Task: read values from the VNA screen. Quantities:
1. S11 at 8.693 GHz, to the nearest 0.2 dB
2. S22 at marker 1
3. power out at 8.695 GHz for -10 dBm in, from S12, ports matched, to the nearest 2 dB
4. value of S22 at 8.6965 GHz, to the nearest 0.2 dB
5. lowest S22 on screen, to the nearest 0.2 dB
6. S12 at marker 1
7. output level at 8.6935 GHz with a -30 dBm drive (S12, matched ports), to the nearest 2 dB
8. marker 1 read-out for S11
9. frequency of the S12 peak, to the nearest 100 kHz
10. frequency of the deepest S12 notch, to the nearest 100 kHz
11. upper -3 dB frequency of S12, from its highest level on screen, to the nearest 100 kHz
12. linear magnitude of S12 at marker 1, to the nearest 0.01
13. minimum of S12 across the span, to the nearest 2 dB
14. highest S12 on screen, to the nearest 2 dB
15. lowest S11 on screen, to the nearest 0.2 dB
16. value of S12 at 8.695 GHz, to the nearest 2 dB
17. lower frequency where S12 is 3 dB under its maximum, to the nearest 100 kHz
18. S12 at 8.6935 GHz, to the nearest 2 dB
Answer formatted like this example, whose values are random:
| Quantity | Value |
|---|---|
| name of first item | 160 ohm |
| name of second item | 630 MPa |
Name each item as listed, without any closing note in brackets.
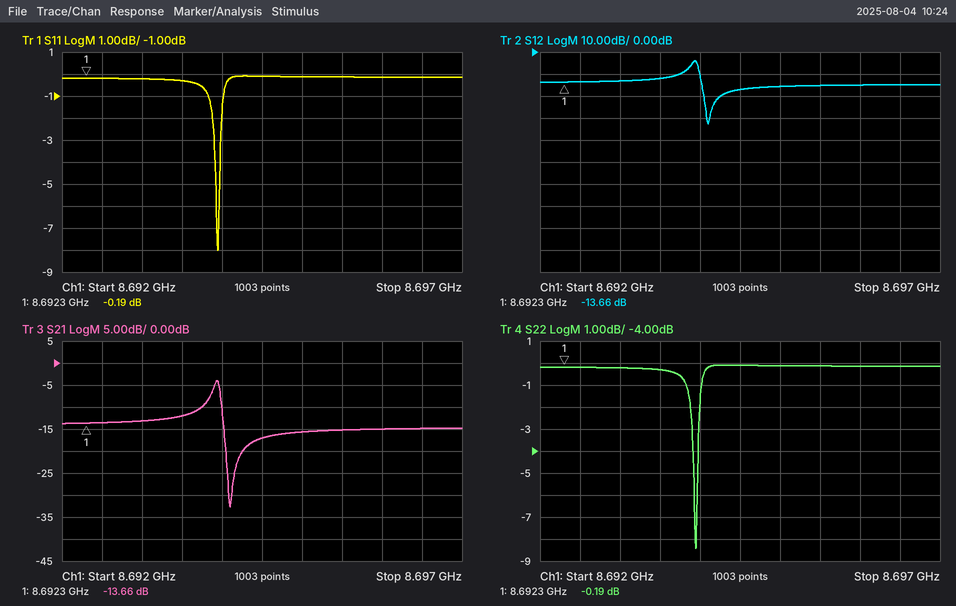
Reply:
| Quantity | Value |
|---|---|
| S11 at 8.693 GHz, to the nearest 0.2 dB | -0.2 dB |
| S22 at marker 1 | -0.19 dB |
| power out at 8.695 GHz for -10 dBm in, from S12, ports matched, to the nearest 2 dB | -26 dBm |
| value of S22 at 8.6965 GHz, to the nearest 0.2 dB | -0.2 dB |
| lowest S22 on screen, to the nearest 0.2 dB | -8.4 dB |
| S12 at marker 1 | -13.66 dB |
| output level at 8.6935 GHz with a -30 dBm drive (S12, matched ports), to the nearest 2 dB | -42 dBm |
| marker 1 read-out for S11 | -0.19 dB |
| frequency of the S12 peak, to the nearest 100 kHz | 8.6939 GHz |
| frequency of the deepest S12 notch, to the nearest 100 kHz | 8.6941 GHz |
| upper -3 dB frequency of S12, from its highest level on screen, to the nearest 100 kHz | 8.6940 GHz |
| linear magnitude of S12 at marker 1, to the nearest 0.01 | 0.21 |
| minimum of S12 across the span, to the nearest 2 dB | -32 dB |
| highest S12 on screen, to the nearest 2 dB | -4 dB |
| lowest S11 on screen, to the nearest 0.2 dB | -8.0 dB |
| value of S12 at 8.695 GHz, to the nearest 2 dB | -16 dB |
| lower frequency where S12 is 3 dB under its maximum, to the nearest 100 kHz | 8.6939 GHz |
| S12 at 8.6935 GHz, to the nearest 2 dB | -12 dB |
